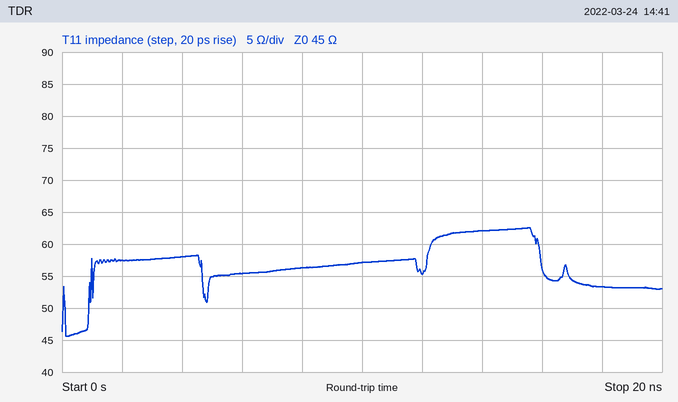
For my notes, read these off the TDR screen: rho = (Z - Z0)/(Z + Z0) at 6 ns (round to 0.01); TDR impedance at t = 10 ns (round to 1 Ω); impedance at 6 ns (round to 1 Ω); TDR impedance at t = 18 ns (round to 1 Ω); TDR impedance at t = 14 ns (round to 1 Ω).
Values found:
+0.10
57 Ω
55 Ω
53 Ω
62 Ω
